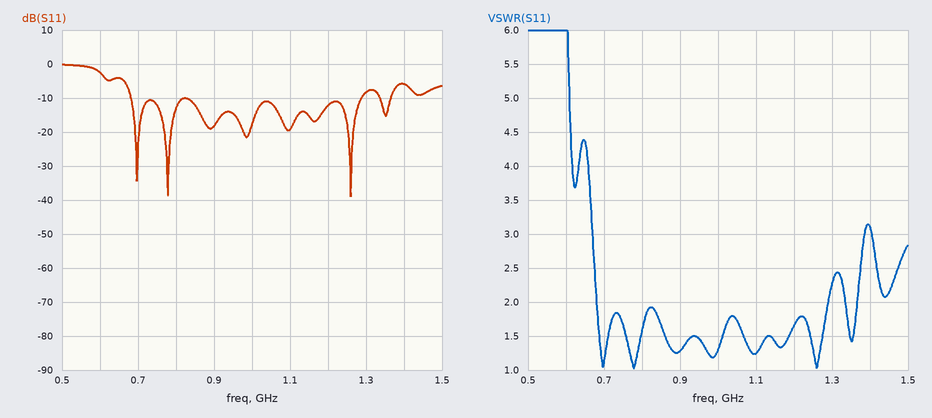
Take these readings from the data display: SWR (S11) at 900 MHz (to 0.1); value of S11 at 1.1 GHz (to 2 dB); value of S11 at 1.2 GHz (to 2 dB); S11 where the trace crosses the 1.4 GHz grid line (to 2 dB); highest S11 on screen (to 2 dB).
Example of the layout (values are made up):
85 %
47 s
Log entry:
1.3
-20 dB
-12 dB
-6 dB
0 dB
